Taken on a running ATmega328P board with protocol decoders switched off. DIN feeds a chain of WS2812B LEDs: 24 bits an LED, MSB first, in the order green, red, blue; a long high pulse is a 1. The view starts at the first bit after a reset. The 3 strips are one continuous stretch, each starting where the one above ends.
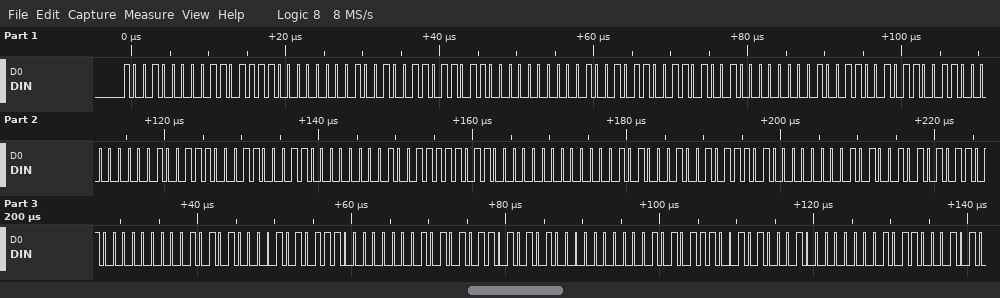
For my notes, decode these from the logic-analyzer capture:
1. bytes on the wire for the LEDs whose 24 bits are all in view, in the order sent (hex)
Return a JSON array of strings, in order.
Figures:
["90 6F 00 93 6C 00 96 69 00 99 66 00 9C 63 00 9F 60 00 A2 5D 00 A5 5A 00 A8 57 00 AB 54 00 AE 51 00"]
